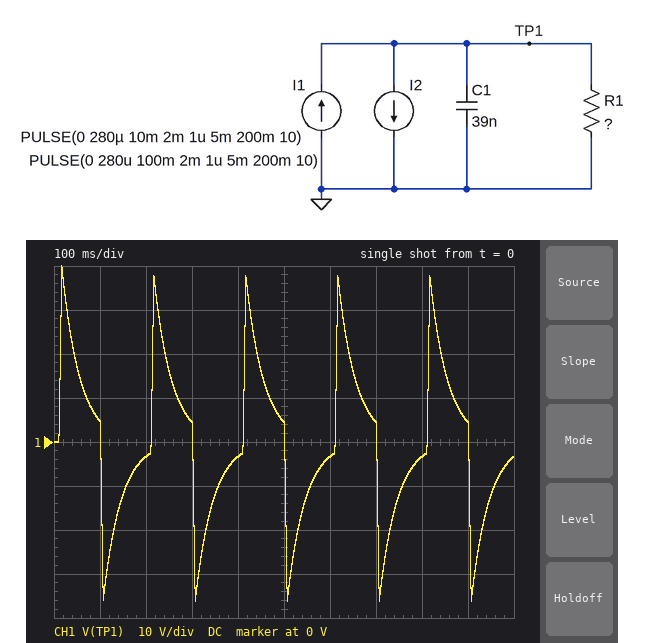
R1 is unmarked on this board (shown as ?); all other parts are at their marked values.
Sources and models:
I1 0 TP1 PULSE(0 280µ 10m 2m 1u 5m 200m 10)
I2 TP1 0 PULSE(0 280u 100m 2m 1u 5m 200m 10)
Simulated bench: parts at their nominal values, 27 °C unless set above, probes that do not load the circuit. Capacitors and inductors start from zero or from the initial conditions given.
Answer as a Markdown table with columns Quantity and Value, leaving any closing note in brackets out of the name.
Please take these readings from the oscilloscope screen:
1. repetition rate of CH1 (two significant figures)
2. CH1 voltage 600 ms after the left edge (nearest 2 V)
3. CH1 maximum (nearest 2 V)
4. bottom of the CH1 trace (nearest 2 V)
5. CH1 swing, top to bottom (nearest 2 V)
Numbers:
| Quantity | Value |
|---|---|
| repetition rate of CH1 | 5.0 Hz |
| CH1 voltage 600 ms after the left edge | -4 V |
| CH1 maximum | 40 V |
| bottom of the CH1 trace | -36 V |
| CH1 swing, top to bottom | 76 V |
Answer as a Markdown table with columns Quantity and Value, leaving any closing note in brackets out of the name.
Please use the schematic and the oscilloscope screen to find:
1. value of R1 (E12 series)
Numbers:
| Quantity | Value |
|---|---|
| value of R1 | 1 MΩ |
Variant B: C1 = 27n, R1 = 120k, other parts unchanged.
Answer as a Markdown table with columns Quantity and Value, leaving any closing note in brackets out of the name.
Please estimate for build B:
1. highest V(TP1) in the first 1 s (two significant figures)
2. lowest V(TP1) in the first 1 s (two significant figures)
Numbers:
| Quantity | Value |
|---|---|
| highest V(TP1) in the first 1 s | 28 V |
| lowest V(TP1) in the first 1 s | -28 V |
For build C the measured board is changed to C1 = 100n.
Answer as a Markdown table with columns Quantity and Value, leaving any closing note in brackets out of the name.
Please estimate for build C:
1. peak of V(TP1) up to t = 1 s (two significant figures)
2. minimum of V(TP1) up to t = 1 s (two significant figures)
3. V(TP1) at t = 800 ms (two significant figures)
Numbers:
| Quantity | Value |
|---|---|
| peak of V(TP1) up to t = 1 s | 16 V |
| minimum of V(TP1) up to t = 1 s | -11 V |
| V(TP1) at t = 800 ms | -4.4 V |
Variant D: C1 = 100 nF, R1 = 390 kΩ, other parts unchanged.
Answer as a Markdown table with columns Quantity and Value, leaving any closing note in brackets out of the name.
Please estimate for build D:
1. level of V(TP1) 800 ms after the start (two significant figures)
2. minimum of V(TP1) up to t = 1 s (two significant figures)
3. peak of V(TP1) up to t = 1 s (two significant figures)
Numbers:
| Quantity | Value |
|---|---|
| level of V(TP1) 800 ms after the start | -1.3 V |
| minimum of V(TP1) up to t = 1 s | -14 V |
| peak of V(TP1) up to t = 1 s | 16 V |
